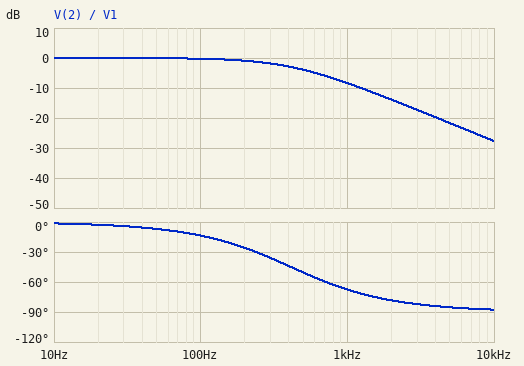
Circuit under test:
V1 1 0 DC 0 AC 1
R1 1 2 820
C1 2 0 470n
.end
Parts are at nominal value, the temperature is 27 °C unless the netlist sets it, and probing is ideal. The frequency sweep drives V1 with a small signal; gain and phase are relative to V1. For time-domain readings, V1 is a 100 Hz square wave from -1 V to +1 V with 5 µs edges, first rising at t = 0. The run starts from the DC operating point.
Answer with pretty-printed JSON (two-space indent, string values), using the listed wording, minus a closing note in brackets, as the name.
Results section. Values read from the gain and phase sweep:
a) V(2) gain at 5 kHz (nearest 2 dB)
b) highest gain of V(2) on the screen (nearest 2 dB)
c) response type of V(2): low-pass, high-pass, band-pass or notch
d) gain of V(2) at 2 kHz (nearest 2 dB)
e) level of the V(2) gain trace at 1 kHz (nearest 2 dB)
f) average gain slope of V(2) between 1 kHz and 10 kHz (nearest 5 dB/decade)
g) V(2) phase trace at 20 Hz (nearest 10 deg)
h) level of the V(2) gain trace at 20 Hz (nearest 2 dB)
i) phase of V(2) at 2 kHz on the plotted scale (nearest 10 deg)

{
  "V(2) gain at 5 kHz": "-22 dB",
  "highest gain of V(2) on the screen": "0 dB",
  "response type of V(2): low-pass, high-pass, band-pass or notch": "low-pass",
  "gain of V(2) at 2 kHz": "-14 dB",
  "level of the V(2) gain trace at 1 kHz": "-8 dB",
  "average gain slope of V(2) between 1 kHz and 10 kHz": "-20 dB/decade",
  "V(2) phase trace at 20 Hz": "0 deg",
  "level of the V(2) gain trace at 20 Hz": "0 dB",
  "phase of V(2) at 2 kHz on the plotted scale": "-80 deg"
}
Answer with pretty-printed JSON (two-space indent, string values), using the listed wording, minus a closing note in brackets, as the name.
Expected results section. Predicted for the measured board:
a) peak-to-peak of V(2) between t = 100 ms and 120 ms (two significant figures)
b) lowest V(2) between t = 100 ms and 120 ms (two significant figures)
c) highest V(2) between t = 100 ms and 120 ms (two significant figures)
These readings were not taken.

{
  "peak-to-peak of V(2) between t = 100 ms and 120 ms": "2.0 V",
  "lowest V(2) between t = 100 ms and 120 ms": "-1.0 V",
  "highest V(2) between t = 100 ms and 120 ms": "1.0 V"
}
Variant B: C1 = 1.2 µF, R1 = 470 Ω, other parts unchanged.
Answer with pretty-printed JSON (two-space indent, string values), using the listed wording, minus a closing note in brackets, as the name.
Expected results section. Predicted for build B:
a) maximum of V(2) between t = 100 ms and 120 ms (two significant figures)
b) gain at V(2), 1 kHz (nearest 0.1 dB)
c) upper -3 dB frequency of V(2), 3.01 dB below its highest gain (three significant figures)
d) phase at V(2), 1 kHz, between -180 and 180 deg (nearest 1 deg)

{
  "maximum of V(2) between t = 100 ms and 120 ms": "1.0 V",
  "gain at V(2), 1 kHz": "-11.3 dB",
  "upper -3 dB frequency of V(2), 3.01 dB below its highest gain": "282 Hz",
  "phase at V(2), 1 kHz, between -180 and 180 deg": "-74 deg"
}
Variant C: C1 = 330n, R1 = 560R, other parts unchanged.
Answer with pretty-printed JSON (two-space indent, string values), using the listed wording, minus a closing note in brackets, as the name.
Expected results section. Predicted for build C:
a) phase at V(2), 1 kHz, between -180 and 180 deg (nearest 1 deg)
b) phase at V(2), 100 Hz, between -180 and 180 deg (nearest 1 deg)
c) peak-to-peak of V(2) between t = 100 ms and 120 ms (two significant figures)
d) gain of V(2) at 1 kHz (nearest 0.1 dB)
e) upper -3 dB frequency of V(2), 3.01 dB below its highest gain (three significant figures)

{
  "phase at V(2), 1 kHz, between -180 and 180 deg": "-49 deg",
  "phase at V(2), 100 Hz, between -180 and 180 deg": "-7 deg",
  "peak-to-peak of V(2) between t = 100 ms and 120 ms": "2.0 V",
  "gain of V(2) at 1 kHz": "-3.7 dB",
  "upper -3 dB frequency of V(2), 3.01 dB below its highest gain": "861 Hz"
}
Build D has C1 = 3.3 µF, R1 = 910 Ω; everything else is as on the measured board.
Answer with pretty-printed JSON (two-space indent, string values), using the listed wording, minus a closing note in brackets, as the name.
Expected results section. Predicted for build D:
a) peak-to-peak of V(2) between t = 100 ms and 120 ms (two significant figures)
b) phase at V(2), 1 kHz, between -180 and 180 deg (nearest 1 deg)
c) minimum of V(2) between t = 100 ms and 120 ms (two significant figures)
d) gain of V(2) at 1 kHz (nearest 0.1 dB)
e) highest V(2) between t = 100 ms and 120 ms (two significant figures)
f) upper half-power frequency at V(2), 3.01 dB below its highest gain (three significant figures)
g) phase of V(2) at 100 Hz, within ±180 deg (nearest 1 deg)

{
  "peak-to-peak of V(2) between t = 100 ms and 120 ms": "1.4 V",
  "phase at V(2), 1 kHz, between -180 and 180 deg": "-87 deg",
  "minimum of V(2) between t = 100 ms and 120 ms": "-680 mV",
  "gain of V(2) at 1 kHz": "-25.5 dB",
  "highest V(2) between t = 100 ms and 120 ms": "680 mV",
  "upper half-power frequency at V(2), 3.01 dB below its highest gain": "53.0 Hz",
  "phase of V(2) at 100 Hz, within ±180 deg": "-62 deg"
}
